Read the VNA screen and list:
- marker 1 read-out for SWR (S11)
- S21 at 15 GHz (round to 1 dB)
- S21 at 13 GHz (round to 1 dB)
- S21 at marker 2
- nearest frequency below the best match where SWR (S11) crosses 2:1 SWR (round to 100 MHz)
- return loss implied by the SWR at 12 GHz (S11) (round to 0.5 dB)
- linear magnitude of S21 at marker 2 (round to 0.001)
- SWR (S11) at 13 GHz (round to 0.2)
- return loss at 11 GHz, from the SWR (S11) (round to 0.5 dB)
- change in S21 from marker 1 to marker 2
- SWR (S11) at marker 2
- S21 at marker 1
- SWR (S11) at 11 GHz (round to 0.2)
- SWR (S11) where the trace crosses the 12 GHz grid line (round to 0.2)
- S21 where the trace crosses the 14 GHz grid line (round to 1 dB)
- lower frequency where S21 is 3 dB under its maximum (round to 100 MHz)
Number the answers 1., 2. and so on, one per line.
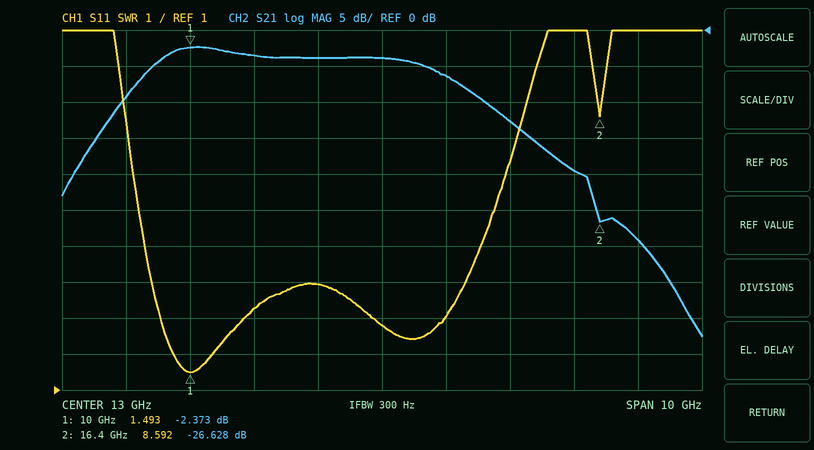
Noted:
1. 1.493
2. -13 dB
3. -4 dB
4. -26.628 dB
5. 9.7 GHz
6. 4.5 dB
7. 0.047
8. 2.8
9. 5.5 dB
10. -24.255 dB
11. 8.592
12. -2.373 dB
13. 3.2
14. 4.0
15. -6 dB
16. 9.4 GHz
